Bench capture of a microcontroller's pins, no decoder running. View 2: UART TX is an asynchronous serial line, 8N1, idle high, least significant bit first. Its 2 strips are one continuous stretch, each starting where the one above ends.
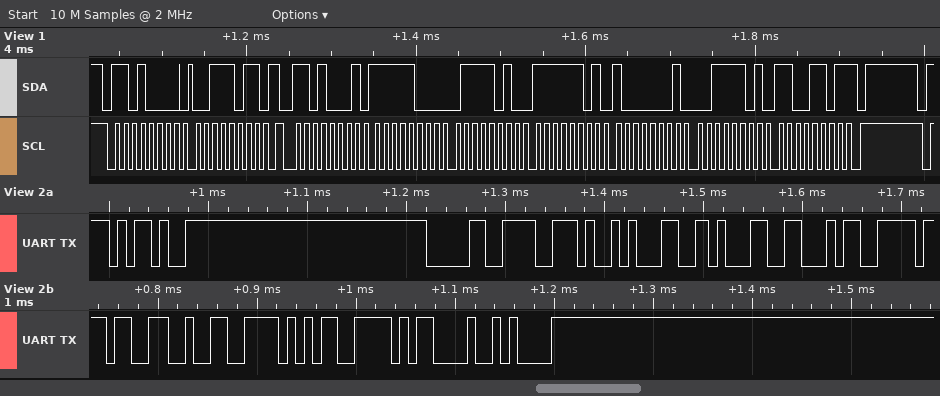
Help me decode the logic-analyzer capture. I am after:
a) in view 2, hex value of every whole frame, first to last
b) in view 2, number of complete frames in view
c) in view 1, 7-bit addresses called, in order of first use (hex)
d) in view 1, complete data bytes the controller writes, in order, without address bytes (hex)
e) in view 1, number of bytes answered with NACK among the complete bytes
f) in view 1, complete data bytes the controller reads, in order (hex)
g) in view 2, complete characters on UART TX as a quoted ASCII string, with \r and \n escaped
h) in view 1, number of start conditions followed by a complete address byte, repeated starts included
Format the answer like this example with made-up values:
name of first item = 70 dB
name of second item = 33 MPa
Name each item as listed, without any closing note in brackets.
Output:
in view 2, hex value of every whole frame, first to last = 0x2D 0x30 0x2E 0x31 0x31 0x34 0x37 0x32 0x35 0x0D 0x0A
in view 2, number of complete frames in view = 11
in view 1, 7-bit addresses called, in order of first use = 0x68
in view 1, complete data bytes the controller writes, in order, without address bytes = 3B
in view 1, number of bytes answered with NACK among the complete bytes = 1
in view 1, complete data bytes the controller reads, in order = F8 7A FD 81 3D CD
in view 2, complete characters on UART TX as a quoted ASCII string, with \r and \n escaped = "-0.114725\r\n"
in view 1, number of start conditions followed by a complete address byte, repeated starts included = 2
